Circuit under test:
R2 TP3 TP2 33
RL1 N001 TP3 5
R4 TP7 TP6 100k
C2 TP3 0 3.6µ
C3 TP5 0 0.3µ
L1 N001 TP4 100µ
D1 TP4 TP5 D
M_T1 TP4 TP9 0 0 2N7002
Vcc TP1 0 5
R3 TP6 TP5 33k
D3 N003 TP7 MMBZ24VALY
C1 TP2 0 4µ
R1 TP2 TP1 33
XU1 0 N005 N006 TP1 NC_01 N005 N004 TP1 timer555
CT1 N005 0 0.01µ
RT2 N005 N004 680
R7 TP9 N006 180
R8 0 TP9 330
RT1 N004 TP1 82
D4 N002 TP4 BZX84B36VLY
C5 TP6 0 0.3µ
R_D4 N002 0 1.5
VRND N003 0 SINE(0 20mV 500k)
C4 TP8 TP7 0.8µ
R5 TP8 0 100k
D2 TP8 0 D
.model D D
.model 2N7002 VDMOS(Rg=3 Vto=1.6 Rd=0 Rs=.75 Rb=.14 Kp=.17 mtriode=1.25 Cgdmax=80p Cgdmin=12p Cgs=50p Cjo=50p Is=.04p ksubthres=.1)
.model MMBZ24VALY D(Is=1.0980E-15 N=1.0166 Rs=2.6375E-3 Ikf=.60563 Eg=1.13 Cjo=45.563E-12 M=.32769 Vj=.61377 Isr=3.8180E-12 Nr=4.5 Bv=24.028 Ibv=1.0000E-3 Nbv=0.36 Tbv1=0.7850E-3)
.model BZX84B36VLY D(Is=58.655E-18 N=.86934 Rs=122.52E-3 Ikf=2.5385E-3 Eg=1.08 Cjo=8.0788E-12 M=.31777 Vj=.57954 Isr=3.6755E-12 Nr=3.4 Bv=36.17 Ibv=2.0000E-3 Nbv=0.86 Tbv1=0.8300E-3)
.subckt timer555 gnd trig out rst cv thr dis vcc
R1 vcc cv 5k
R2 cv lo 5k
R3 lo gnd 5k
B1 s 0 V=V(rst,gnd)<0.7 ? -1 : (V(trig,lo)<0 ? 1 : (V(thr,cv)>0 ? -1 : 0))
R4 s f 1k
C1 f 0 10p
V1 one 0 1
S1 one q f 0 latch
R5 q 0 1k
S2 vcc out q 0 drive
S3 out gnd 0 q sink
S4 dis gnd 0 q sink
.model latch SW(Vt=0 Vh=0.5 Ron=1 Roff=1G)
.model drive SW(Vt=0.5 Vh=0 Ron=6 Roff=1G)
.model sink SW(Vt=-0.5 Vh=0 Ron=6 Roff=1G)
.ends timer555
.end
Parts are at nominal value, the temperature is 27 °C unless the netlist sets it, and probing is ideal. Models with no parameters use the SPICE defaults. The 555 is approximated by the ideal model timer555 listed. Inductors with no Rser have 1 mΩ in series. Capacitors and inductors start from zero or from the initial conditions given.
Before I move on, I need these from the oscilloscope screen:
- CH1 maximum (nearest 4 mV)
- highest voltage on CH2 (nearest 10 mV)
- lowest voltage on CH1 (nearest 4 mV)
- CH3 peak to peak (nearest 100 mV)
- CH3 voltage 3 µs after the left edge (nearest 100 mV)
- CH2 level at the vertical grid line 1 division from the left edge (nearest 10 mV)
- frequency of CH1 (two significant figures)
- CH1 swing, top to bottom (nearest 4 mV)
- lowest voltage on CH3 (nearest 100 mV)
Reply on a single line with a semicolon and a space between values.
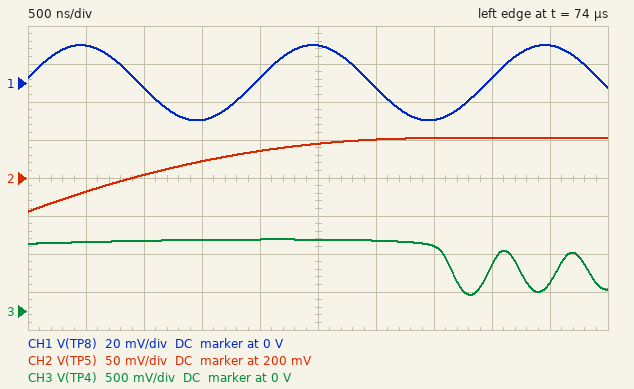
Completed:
20 mV; 250 mV; -20 mV; 700 mV; 900 mV; 180 mV; 500 kHz; 40 mV; 200 mV
